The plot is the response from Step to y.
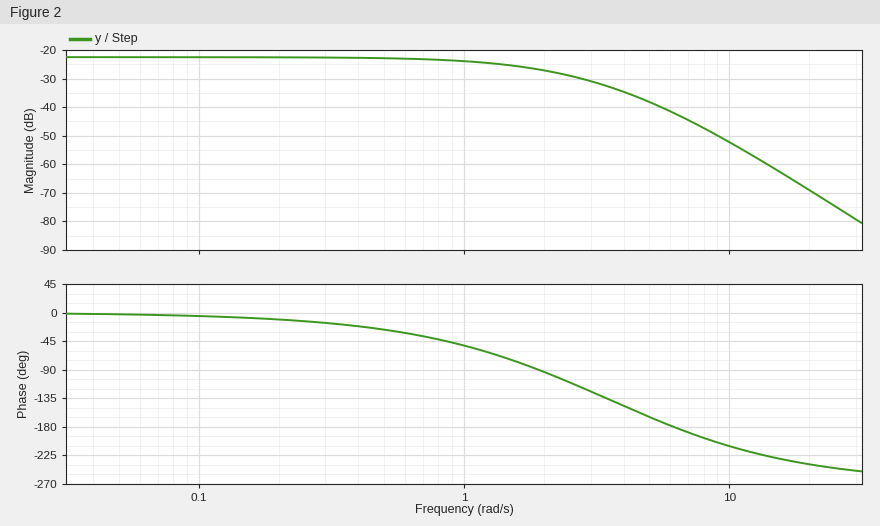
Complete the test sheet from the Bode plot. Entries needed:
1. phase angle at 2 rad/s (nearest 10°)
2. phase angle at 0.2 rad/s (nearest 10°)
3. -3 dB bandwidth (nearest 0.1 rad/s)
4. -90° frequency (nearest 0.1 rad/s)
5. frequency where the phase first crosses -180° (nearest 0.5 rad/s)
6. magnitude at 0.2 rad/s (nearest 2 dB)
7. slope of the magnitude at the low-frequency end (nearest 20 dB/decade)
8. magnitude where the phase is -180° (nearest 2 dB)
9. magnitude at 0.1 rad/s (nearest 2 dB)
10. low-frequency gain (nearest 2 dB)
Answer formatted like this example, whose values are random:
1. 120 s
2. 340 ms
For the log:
1. -90°
2. -10°
3. 1.5 rad/s
4. 1.9 rad/s
5. 6.0 rad/s
6. -22 dB
7. 0 dB/decade
8. -42 dB
9. -22 dB
10. -22 dB
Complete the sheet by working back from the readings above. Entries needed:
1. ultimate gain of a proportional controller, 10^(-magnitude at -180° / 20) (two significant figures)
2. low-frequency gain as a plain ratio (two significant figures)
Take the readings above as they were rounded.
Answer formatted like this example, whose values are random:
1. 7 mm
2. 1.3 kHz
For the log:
1. 130
2. 0.079
